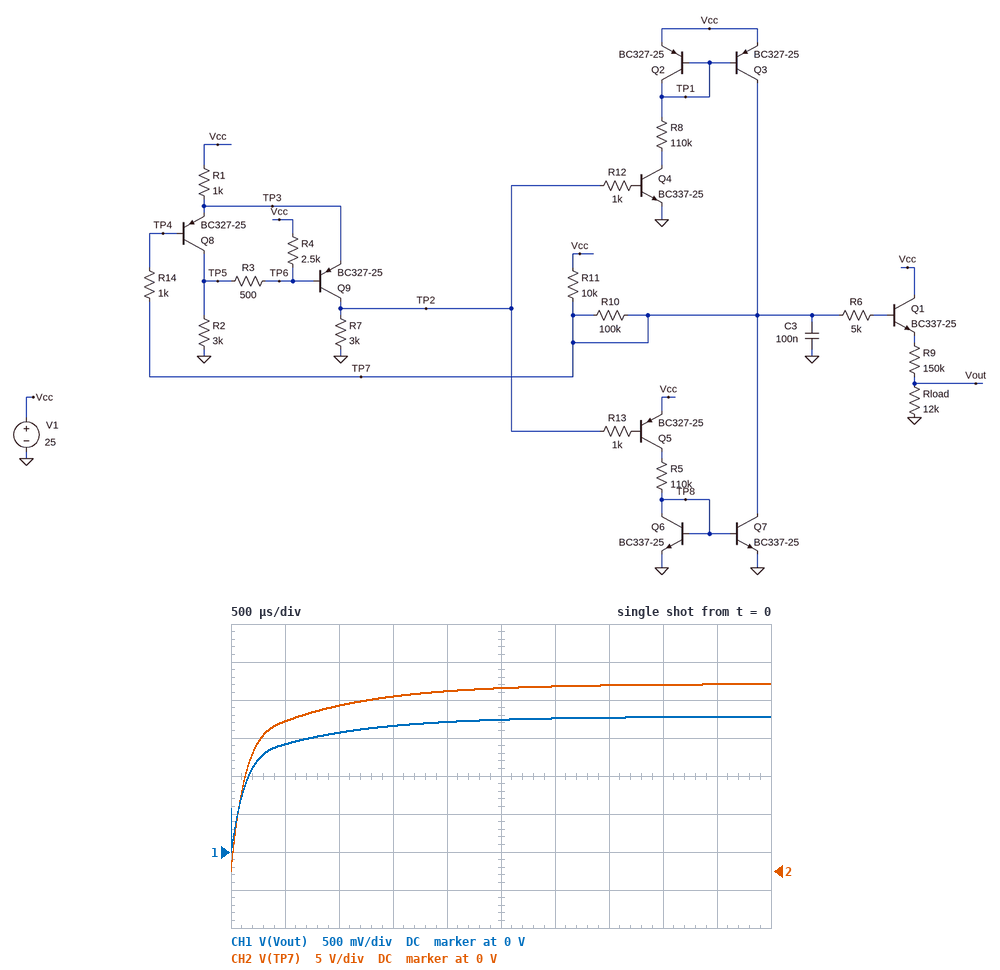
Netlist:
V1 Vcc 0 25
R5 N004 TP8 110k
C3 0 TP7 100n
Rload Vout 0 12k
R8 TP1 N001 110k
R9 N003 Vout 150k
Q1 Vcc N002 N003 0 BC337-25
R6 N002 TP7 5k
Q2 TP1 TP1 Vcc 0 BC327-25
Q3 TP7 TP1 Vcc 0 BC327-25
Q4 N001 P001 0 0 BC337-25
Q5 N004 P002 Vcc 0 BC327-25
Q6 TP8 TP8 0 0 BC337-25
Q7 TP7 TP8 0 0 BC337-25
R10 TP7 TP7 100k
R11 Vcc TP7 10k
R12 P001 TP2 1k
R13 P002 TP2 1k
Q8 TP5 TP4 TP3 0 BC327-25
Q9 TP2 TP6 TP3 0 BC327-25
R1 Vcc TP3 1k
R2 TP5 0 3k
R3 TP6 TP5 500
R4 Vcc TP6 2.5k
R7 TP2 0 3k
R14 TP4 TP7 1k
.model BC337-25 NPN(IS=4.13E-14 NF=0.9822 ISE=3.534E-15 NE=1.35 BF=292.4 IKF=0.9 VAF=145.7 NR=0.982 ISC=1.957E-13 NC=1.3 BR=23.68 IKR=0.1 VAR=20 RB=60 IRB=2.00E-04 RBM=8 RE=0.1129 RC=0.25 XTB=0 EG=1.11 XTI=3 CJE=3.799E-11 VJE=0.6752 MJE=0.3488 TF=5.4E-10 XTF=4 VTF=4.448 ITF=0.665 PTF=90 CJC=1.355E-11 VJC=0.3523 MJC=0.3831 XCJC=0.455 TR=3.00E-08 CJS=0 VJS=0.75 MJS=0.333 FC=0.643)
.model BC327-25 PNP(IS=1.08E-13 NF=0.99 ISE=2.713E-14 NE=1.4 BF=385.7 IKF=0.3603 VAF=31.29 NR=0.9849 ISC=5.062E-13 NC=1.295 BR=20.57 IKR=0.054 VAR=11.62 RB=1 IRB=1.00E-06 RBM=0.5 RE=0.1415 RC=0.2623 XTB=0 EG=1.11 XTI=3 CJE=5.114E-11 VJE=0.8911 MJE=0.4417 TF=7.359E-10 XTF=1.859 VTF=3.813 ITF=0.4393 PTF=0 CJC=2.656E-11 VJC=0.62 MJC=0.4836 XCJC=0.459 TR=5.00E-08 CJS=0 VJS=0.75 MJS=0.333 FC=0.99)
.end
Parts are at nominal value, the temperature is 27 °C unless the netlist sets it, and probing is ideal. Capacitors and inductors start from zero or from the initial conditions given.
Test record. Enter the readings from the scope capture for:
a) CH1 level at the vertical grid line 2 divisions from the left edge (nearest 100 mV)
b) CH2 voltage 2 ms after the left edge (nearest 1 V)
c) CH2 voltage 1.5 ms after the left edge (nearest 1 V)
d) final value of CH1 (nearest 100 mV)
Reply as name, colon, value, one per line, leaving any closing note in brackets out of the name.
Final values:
CH1 level at the vertical grid line 2 divisions from the left edge: 1.6 V
CH2 voltage 2 ms after the left edge: 24 V
CH2 voltage 1.5 ms after the left edge: 23 V
final value of CH1: 1.8 V
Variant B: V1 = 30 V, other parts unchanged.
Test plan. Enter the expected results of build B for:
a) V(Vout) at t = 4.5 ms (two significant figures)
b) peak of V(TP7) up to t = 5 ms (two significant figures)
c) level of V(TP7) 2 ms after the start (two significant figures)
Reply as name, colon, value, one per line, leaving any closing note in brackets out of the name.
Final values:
V(Vout) at t = 4.5 ms: 2.1 V
peak of V(TP7) up to t = 5 ms: 29 V
level of V(TP7) 2 ms after the start: 28 V
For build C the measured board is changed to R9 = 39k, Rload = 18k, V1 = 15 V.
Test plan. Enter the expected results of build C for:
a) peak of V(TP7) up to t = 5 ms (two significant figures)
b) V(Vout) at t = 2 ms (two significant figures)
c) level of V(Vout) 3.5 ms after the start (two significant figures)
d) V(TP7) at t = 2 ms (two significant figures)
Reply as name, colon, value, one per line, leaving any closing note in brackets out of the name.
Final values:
peak of V(TP7) up to t = 5 ms: 15 V
V(Vout) at t = 2 ms: 4.3 V
level of V(Vout) 3.5 ms after the start: 4.5 V
V(TP7) at t = 2 ms: 14 V
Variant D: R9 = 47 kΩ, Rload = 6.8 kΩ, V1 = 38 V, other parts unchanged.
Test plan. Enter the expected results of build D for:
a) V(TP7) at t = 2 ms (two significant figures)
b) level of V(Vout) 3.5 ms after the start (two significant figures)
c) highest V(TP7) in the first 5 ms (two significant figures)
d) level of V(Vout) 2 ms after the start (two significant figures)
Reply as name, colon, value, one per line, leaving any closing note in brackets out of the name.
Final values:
V(TP7) at t = 2 ms: 36 V
level of V(Vout) 3.5 ms after the start: 4.6 V
highest V(TP7) in the first 5 ms: 37 V
level of V(Vout) 2 ms after the start: 4.5 V
